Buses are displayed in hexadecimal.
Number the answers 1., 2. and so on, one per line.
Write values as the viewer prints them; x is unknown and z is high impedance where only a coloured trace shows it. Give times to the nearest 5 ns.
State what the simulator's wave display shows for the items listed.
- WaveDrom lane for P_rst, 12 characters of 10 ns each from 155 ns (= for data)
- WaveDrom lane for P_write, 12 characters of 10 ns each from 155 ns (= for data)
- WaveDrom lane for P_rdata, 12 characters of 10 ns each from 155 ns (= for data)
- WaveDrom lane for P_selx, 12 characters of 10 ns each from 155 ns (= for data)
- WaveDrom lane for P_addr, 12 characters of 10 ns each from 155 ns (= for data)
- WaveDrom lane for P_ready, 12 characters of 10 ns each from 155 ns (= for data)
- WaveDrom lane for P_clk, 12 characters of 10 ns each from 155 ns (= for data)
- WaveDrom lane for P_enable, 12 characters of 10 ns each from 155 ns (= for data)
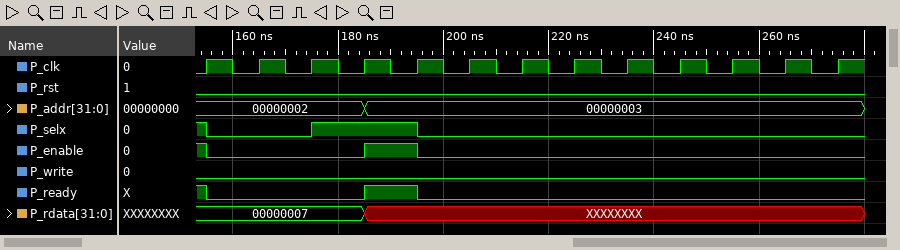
1. {name: 'P_rst', wave: '0...........'}
2. {name: 'P_write', wave: '0...........'}
3. {name: 'P_rdata', wave: '=..x........', data: '00000007'}
4. {name: 'P_selx', wave: '0.1.0.......'}
5. {name: 'P_addr', wave: '=..=........', data: '00000002 00000003'}
6. {name: 'P_ready', wave: '0..10.......'}
7. {name: 'P_clk', wave: 'p...........'}
8. {name: 'P_enable', wave: '0..10.......'}
